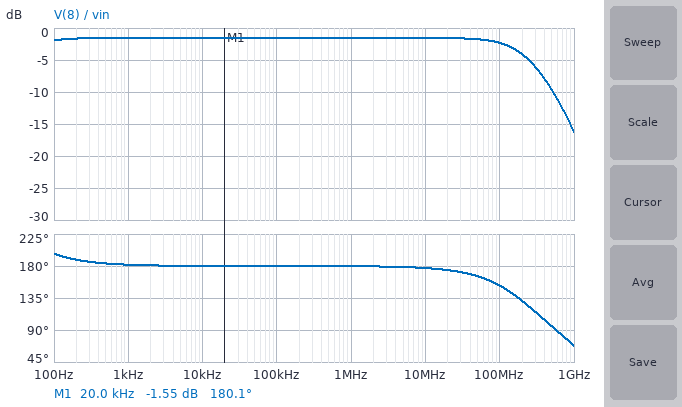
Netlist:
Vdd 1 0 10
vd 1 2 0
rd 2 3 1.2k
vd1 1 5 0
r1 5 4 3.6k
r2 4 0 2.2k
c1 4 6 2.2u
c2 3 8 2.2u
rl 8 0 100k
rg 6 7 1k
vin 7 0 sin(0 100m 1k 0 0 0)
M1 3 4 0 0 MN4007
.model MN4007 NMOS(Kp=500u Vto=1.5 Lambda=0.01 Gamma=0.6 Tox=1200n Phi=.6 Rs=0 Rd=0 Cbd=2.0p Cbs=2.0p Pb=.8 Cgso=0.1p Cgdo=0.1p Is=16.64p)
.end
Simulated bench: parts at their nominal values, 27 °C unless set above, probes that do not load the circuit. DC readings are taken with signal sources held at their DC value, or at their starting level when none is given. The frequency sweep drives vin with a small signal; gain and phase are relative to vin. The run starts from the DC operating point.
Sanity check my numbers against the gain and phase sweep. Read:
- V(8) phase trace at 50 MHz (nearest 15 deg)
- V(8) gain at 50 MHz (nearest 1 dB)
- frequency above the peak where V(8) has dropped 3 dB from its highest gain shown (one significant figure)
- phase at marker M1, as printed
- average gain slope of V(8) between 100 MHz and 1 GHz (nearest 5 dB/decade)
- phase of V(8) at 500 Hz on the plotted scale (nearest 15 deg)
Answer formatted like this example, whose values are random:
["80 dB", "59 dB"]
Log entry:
["165 deg", "-2 dB", "200 MHz", "180.1 deg", "-15 dB/decade", "180 deg"]
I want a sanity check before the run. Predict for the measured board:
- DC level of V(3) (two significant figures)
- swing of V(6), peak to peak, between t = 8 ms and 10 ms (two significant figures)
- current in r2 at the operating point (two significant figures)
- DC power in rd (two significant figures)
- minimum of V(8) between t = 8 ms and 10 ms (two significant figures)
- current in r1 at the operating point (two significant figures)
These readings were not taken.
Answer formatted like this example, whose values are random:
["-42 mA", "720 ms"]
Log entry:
["8.3 V", "120 mV", "1.7 mA", "2.4 mW", "-84 mV", "1.7 mA"]
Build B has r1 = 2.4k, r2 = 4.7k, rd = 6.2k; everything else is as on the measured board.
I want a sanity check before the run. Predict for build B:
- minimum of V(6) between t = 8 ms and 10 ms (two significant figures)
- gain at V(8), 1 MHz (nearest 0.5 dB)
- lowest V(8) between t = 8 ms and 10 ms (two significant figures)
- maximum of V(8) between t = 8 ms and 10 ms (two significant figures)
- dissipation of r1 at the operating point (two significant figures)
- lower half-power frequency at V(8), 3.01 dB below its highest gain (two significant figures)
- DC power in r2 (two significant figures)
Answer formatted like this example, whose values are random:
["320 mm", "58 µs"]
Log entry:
["-61 mV", "-22.0 dB", "-7.7 mV", "8.0 mV", "4.8 mW", "28 Hz", "9.3 mW"]
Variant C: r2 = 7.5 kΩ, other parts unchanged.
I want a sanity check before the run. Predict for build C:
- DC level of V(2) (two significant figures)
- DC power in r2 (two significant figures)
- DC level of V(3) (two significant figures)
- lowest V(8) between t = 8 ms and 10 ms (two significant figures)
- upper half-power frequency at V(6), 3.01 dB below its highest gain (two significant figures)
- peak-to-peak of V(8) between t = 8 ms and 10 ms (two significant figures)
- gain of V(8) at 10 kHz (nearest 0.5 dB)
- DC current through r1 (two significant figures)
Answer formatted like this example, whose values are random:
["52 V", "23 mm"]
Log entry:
["10 V", "6.1 mW", "3.0 V", "-52 mV", "31 MHz", "110 mV", "-5.5 dB", "900 µA"]
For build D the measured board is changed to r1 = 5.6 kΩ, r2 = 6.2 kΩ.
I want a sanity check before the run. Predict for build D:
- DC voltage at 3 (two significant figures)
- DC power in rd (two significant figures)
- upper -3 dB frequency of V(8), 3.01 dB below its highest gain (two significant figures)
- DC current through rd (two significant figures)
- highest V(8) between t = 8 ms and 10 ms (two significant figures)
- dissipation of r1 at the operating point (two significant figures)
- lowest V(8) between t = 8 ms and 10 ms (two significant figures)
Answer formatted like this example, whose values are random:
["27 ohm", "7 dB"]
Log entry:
["5.5 V", "17 mW", "190 MHz", "3.7 mA", "170 mV", "4.0 mW", "-170 mV"]
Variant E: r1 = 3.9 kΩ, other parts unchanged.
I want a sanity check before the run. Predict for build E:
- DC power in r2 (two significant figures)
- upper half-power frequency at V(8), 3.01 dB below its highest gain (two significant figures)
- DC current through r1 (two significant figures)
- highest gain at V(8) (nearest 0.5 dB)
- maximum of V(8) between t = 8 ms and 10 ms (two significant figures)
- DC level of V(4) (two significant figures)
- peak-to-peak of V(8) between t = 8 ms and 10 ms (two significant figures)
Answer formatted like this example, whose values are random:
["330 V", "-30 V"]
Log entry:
["5.9 mW", "230 MHz", "1.6 mA", "-2.0 dB", "78 mV", "3.6 V", "160 mV"]
